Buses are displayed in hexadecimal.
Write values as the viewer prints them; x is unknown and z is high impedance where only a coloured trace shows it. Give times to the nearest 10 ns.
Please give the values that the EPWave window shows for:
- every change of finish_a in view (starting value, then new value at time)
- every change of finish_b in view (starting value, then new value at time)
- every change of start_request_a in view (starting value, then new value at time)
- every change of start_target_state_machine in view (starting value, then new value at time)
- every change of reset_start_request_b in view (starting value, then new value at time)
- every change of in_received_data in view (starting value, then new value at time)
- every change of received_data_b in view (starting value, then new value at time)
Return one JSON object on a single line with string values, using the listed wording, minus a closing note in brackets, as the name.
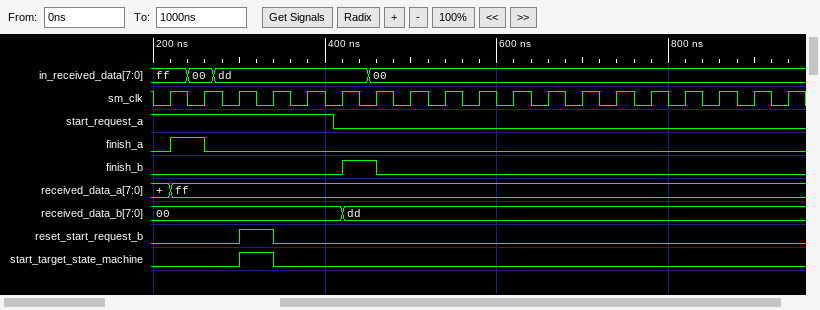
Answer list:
{"every change of finish_a in view": "0, 1 at 220 ns, 0 at 260 ns", "every change of finish_b in view": "0, 1 at 420 ns, 0 at 460 ns", "every change of start_request_a in view": "1, 0 at 410 ns", "every change of start_target_state_machine in view": "0, 1 at 300 ns, 0 at 340 ns", "every change of reset_start_request_b in view": "0, 1 at 300 ns, 0 at 340 ns", "every change of in_received_data in view": "ff, 00 at 240 ns, dd at 270 ns, 00 at 450 ns", "every change of received_data_b in view": "00, dd at 420 ns"}
